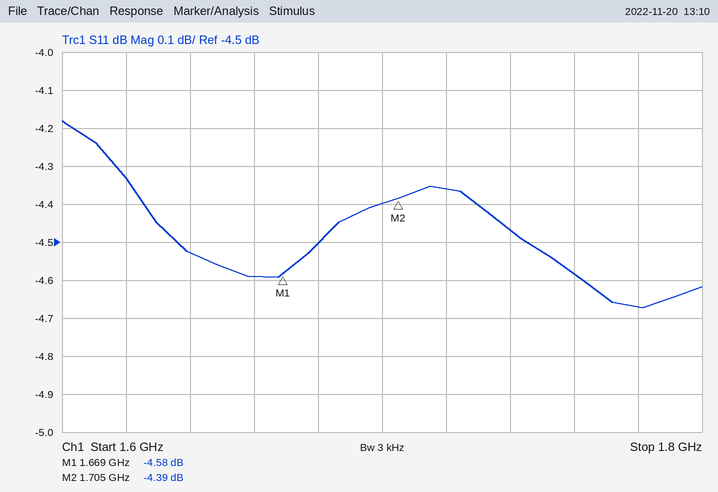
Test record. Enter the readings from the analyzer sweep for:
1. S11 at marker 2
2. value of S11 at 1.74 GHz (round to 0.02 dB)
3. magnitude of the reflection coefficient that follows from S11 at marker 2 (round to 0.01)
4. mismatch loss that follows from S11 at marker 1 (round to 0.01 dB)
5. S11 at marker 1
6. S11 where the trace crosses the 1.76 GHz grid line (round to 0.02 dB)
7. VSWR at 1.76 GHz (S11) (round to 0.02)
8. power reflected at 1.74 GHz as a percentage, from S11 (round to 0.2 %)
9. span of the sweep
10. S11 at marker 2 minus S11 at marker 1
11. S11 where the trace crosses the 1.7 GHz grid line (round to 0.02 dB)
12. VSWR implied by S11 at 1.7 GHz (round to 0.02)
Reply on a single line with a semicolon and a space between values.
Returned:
-4.39 dB; -4.46 dB; 0.60; 1.86 dB; -4.58 dB; -4.58 dB; 3.88; 35.8 %; 200 MHz; 0.19 dB; -4.40 dB; 4.04
